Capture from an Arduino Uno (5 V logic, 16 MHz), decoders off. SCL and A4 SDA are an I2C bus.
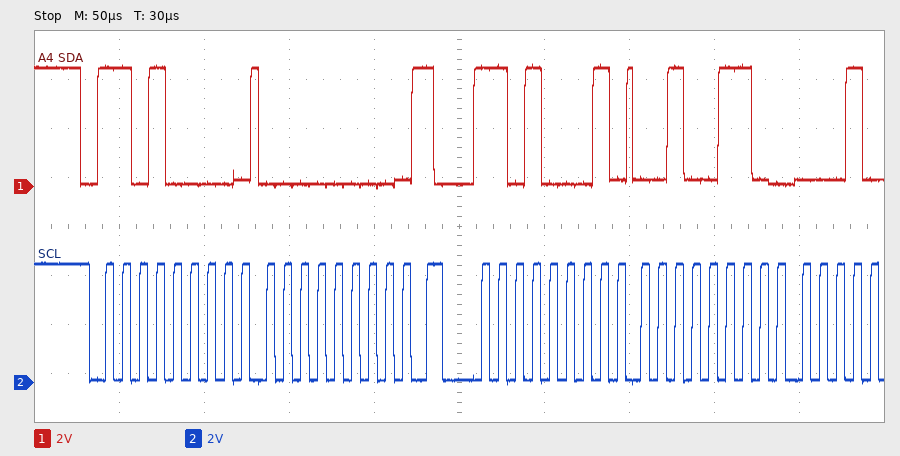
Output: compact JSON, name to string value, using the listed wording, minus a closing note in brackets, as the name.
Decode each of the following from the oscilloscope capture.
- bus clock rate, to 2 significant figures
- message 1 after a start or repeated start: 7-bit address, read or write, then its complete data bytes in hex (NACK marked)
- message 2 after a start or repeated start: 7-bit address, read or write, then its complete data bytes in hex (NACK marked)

{"bus clock rate, to 2 significant figures": "100 kHz", "message 1 after a start or repeated start: 7-bit address, read or write, then its complete data bytes in hex": "0x68 write: 00", "message 2 after a start or repeated start: 7-bit address, read or write, then its complete data bytes in hex": "0x68 read: 26"}
